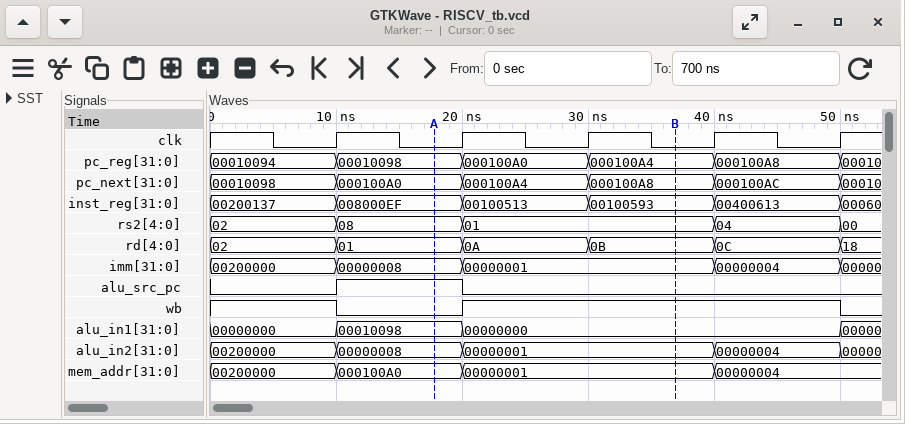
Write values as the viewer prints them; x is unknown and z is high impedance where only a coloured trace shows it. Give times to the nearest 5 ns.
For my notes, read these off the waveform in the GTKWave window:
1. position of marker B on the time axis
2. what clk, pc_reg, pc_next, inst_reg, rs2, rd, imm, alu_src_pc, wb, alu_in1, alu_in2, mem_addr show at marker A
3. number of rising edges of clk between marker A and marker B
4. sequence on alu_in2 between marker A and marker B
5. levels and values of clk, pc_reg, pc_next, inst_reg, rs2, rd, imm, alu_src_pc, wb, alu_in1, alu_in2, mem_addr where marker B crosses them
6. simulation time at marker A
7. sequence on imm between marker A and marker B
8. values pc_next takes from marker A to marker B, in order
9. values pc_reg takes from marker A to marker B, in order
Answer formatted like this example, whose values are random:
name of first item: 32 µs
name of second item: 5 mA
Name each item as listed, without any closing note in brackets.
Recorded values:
position of marker B on the time axis: 35 ns
what clk, pc_reg, pc_next, inst_reg, rs2, rd, imm, alu_src_pc, wb, alu_in1, alu_in2, mem_addr show at marker A: clk=0, pc_reg=00010098, pc_next=000100A0, inst_reg=008000EF, rs2=08, rd=01, imm=00000008, alu_src_pc=1, wb=0, alu_in1=00010098, alu_in2=00000008, mem_addr=000100A0
number of rising edges of clk between marker A and marker B: 2
sequence on alu_in2 between marker A and marker B: 00000008, 00000001
levels and values of clk, pc_reg, pc_next, inst_reg, rs2, rd, imm, alu_src_pc, wb, alu_in1, alu_in2, mem_addr where marker B crosses them: clk=0, pc_reg=000100A4, pc_next=000100A8, inst_reg=00100593, rs2=01, rd=0B, imm=00000001, alu_src_pc=0, wb=1, alu_in1=00000000, alu_in2=00000001, mem_addr=00000001
simulation time at marker A: 20 ns
sequence on imm between marker A and marker B: 00000008, 00000001
values pc_next takes from marker A to marker B, in order: 000100A0, 000100A4, 000100A8
values pc_reg takes from marker A to marker B, in order: 00010098, 000100A0, 000100A4
